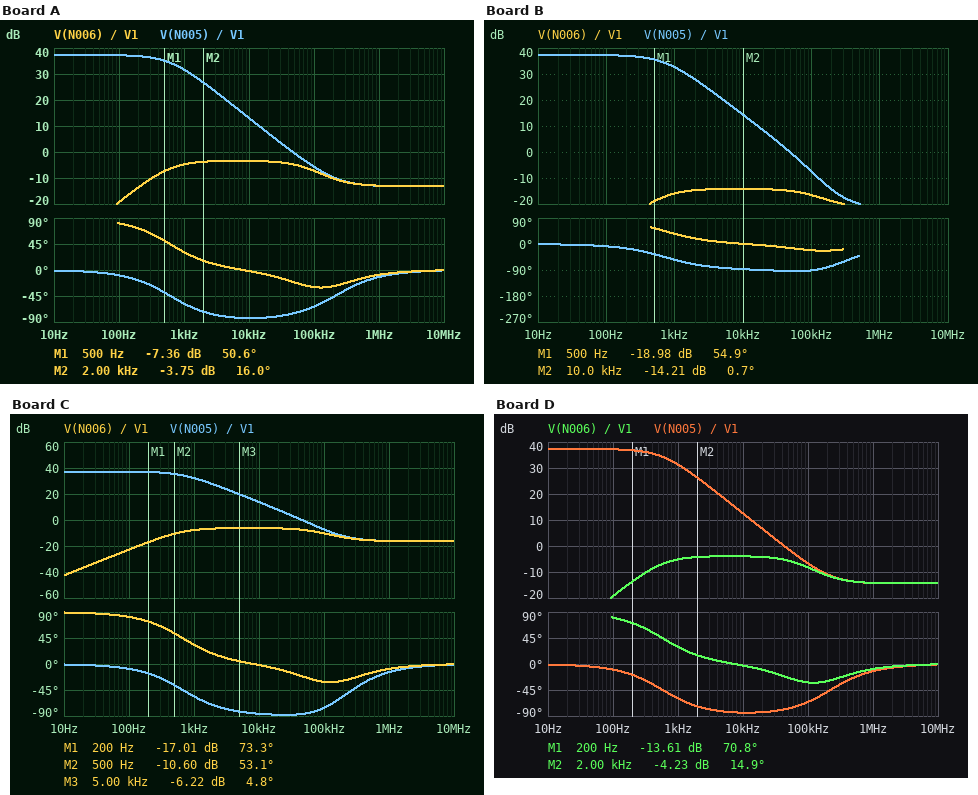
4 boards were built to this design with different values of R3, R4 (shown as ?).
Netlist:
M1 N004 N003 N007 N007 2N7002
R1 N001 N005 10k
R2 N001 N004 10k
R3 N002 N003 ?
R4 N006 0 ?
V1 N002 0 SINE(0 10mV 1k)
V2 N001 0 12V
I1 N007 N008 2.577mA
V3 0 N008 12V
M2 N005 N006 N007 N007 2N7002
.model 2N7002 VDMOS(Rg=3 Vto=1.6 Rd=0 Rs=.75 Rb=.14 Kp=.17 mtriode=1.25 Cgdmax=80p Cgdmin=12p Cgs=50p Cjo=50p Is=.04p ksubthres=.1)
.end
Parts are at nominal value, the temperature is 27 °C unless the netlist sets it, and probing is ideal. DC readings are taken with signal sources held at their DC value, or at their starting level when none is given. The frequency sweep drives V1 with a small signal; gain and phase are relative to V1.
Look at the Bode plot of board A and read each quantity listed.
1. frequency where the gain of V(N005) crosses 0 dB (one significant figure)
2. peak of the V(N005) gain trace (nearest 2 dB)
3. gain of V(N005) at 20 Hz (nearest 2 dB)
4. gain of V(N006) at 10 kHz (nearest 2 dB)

50 kHz
38 dB
38 dB
-4 dB
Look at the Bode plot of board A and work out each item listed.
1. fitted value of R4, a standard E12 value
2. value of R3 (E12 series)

33 kΩ
15 kΩ
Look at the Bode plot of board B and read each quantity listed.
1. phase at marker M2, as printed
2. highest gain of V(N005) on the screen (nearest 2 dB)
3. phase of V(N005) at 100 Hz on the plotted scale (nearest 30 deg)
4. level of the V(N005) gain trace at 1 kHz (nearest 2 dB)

0.7 deg
38 dB
0 deg
32 dB
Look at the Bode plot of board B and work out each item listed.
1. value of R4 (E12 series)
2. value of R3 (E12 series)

8.2 kΩ
33 kΩ
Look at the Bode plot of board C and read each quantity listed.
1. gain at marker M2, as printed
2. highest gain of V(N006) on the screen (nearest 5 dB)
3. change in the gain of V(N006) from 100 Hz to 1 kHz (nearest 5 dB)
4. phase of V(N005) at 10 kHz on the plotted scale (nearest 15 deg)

-10.60 dB
-5 dB
15 dB
-90 deg
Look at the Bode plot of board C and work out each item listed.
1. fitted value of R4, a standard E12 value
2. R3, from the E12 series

22 kΩ
22 kΩ
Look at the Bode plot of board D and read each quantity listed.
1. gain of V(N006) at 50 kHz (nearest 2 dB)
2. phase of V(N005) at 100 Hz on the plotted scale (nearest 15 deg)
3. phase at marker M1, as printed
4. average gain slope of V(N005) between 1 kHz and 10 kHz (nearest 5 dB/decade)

-6 dB
-15 deg
70.8 deg
-20 dB/decade
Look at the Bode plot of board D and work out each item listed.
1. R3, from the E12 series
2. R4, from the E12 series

18 kΩ
33 kΩ
